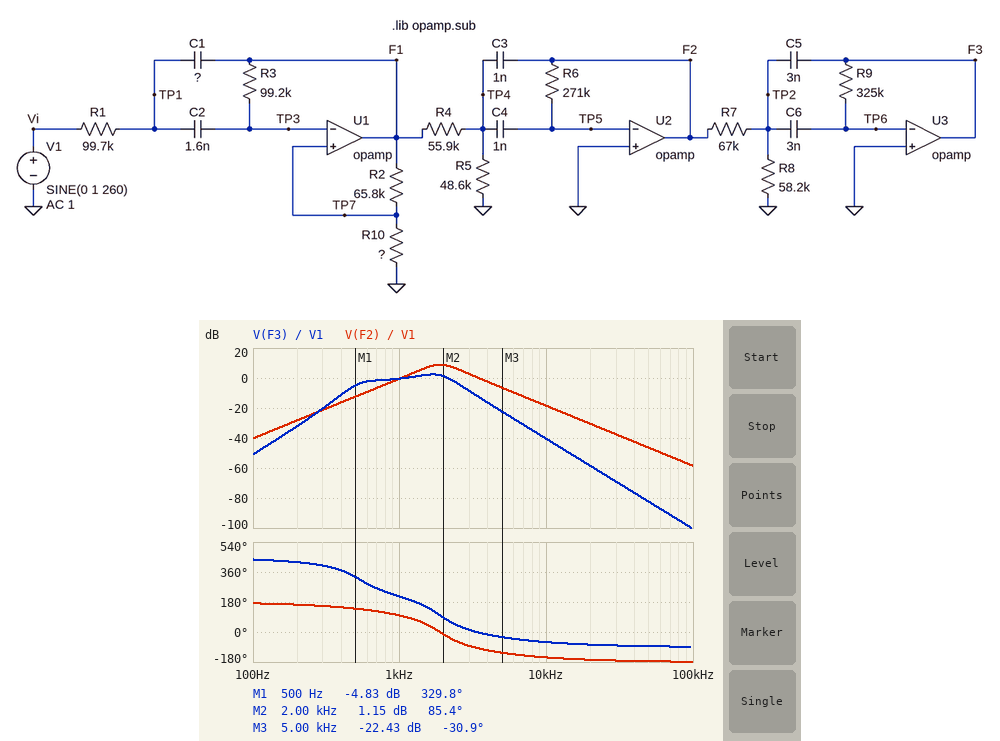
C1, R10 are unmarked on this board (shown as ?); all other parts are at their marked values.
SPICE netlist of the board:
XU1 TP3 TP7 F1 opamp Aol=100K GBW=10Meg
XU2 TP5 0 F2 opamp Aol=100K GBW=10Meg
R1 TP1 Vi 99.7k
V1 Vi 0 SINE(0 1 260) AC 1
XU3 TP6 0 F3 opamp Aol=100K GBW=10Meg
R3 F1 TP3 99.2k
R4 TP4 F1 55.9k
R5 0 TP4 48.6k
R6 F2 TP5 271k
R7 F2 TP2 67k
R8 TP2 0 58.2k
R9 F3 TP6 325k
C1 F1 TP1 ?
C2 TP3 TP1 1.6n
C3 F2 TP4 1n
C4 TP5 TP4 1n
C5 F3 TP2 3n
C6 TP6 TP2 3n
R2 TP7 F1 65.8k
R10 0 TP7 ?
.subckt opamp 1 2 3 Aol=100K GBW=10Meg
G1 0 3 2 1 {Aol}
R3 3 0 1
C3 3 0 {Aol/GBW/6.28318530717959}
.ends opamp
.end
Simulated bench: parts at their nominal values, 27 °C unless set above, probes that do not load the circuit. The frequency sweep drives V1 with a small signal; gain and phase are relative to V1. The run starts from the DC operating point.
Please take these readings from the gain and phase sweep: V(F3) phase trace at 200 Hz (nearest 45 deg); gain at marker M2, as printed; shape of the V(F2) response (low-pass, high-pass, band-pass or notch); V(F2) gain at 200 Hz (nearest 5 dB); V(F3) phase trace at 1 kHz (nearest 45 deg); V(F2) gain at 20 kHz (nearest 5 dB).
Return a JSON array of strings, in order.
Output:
["405 deg", "1.15 dB", "band-pass", "-30 dB", "225 deg", "-30 dB"]
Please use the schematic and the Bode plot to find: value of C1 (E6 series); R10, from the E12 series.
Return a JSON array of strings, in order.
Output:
["470 pF", "15 kΩ"]
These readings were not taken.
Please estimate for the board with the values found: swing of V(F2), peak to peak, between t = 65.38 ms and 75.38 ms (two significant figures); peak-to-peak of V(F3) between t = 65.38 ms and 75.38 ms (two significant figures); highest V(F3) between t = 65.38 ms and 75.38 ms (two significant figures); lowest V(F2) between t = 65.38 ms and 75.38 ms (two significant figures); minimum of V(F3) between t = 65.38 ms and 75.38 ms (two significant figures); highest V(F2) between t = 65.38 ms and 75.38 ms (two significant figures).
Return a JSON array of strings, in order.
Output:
["130 mV", "120 mV", "59 mV", "-65 mV", "-59 mV", "65 mV"]
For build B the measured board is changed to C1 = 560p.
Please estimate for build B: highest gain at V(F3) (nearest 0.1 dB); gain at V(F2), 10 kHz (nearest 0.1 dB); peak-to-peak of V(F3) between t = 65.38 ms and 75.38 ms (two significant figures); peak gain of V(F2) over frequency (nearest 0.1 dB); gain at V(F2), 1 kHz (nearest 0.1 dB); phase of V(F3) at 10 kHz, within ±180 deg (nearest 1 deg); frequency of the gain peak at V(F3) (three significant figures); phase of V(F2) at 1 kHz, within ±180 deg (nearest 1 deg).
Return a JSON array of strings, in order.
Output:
["2.0 dB", "-20.0 dB", "120 mV", "8.4 dB", "-0.5 dB", "-63 deg", "1.67 kHz", "96 deg"]
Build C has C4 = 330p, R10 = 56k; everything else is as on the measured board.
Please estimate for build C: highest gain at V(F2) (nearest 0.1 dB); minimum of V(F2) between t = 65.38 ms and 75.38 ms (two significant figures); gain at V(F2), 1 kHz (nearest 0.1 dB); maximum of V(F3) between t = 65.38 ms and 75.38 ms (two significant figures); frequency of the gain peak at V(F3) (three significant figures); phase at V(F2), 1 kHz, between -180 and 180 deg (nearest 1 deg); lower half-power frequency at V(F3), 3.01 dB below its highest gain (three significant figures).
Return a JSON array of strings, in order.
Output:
["9.9 dB", "-33 mV", "-4.2 dB", "30 mV", "1.96 kHz", "134 deg", "1.28 kHz"]
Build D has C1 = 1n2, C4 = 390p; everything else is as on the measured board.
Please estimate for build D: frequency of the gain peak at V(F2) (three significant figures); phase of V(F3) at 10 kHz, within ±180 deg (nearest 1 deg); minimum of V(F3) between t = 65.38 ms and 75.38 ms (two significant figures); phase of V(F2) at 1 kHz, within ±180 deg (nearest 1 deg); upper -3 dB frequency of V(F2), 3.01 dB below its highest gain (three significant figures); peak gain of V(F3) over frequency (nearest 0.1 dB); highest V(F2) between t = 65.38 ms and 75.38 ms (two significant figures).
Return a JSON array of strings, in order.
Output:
["2.74 kHz", "-64 deg", "-23 mV", "85 deg", "3.69 kHz", "-11.2 dB", "25 mV"]
